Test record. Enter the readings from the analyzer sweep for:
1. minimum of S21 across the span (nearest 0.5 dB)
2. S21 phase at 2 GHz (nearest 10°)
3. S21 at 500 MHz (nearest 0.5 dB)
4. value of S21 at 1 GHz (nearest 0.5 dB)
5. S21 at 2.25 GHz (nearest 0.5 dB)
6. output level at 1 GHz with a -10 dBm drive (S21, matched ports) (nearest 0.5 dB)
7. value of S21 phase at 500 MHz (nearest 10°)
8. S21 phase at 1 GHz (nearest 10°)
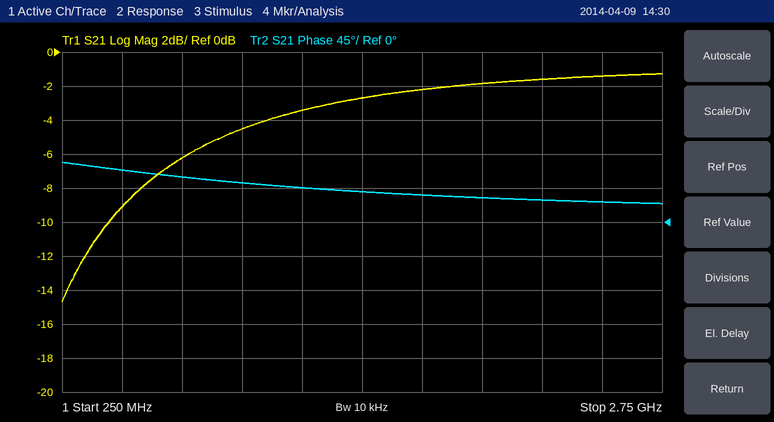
-14.5 dB
30°
-9.0 dB
-4.5 dB
-1.5 dB
-14.5 dBm
70°
50°
